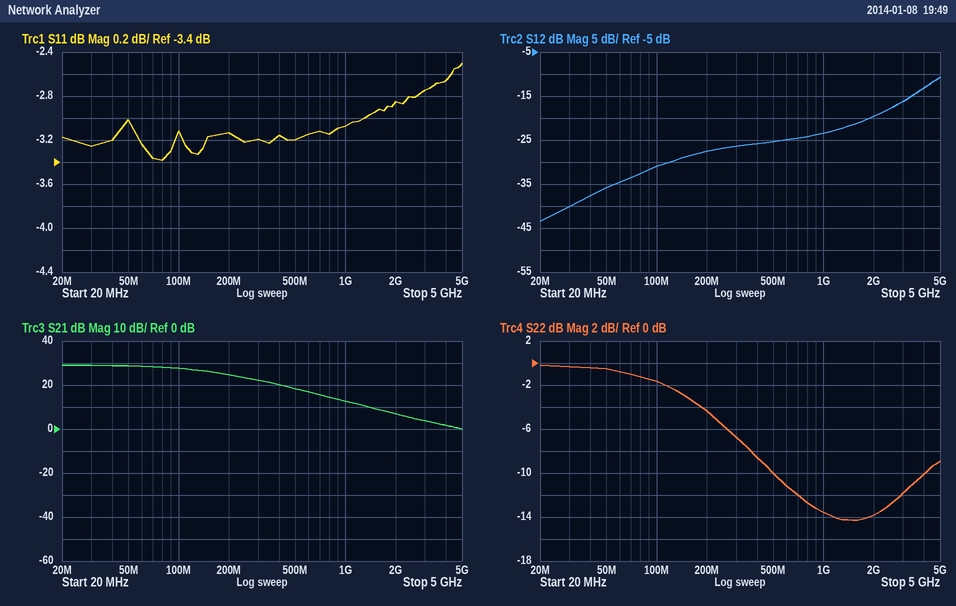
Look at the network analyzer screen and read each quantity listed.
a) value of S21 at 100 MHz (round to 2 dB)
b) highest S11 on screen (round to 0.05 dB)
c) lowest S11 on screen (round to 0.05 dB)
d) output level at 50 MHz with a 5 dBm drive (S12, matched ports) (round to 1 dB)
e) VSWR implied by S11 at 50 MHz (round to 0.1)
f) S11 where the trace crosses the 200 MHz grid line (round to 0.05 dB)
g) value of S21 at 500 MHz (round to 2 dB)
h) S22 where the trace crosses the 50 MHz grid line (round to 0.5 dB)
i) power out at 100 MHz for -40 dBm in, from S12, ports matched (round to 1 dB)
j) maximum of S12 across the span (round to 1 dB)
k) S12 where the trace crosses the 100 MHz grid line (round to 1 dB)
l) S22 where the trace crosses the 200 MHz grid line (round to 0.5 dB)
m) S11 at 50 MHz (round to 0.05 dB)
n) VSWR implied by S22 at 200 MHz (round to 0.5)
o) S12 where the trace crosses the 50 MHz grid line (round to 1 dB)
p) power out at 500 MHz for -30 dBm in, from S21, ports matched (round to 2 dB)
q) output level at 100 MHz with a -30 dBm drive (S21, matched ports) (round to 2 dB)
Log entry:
28 dB
-2.50 dB
-3.40 dB
-31 dBm
5.8
-3.15 dB
18 dB
-0.5 dB
-71 dBm
-11 dB
-31 dB
-4.5 dB
-3.00 dB
4.0
-36 dB
-12 dBm
-2 dBm
